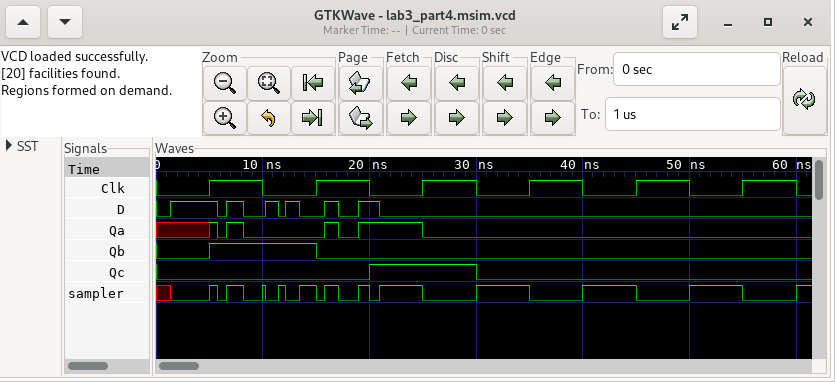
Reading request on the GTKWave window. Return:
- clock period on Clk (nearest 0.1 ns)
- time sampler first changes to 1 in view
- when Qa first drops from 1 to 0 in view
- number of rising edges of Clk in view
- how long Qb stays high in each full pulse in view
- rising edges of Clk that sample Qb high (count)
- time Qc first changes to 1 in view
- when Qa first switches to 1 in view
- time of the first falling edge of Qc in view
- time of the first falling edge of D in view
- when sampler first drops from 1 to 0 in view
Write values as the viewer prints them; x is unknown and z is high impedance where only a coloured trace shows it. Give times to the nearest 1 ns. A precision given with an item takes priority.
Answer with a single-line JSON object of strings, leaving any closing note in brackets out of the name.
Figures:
{"clock period on Clk": "10 ns", "time sampler first changes to 1 in view": "5 ns", "when Qa first drops from 1 to 0 in view": "6 ns", "number of rising edges of Clk in view": "6", "how long Qb stays high in each full pulse in view": "10 ns", "rising edges of Clk that sample Qb high": "1", "time Qc first changes to 1 in view": "20 ns", "when Qa first switches to 1 in view": "5 ns", "time of the first falling edge of Qc in view": "30 ns", "time of the first falling edge of D in view": "6 ns", "when sampler first drops from 1 to 0 in view": "6 ns"}
